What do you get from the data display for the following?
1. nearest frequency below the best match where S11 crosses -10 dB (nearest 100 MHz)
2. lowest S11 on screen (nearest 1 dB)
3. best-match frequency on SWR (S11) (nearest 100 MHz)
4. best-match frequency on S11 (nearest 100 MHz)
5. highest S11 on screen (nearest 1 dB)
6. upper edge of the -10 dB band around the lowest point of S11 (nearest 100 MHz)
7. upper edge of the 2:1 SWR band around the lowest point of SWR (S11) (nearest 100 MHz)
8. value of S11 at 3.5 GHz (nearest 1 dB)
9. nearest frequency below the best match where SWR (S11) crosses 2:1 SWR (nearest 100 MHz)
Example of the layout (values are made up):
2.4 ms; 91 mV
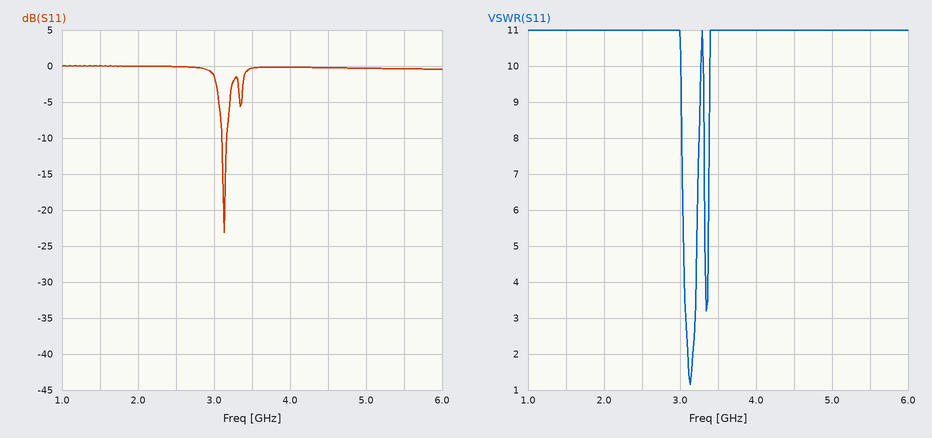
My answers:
3.1 GHz; -23 dB; 3.1 GHz; 3.1 GHz; 0 dB; 3.2 GHz; 3.2 GHz; 0 dB; 3.1 GHz
